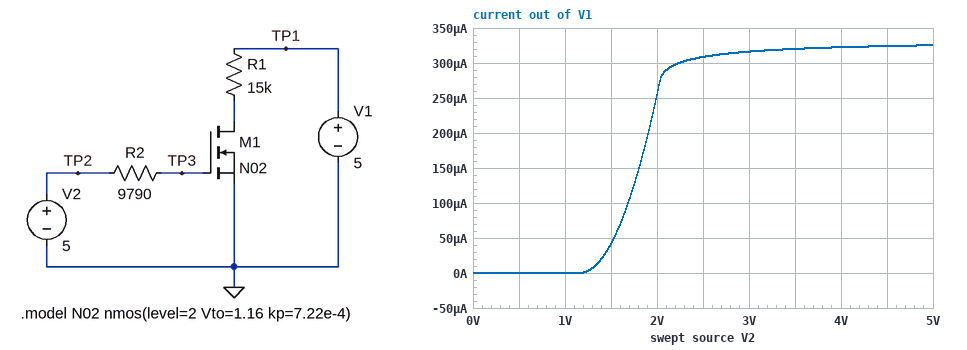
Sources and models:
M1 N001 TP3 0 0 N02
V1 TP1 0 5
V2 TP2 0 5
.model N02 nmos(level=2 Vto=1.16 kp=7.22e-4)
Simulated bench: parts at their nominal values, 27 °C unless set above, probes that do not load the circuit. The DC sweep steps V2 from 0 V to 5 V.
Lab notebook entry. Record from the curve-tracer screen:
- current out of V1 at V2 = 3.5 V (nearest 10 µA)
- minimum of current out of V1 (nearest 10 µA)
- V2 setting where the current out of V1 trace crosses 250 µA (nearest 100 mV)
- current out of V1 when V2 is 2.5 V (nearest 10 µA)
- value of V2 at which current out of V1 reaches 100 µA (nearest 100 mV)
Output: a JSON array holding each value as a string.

["320 µA", "0 A", "2.0 V", "310 µA", "1.7 V"]
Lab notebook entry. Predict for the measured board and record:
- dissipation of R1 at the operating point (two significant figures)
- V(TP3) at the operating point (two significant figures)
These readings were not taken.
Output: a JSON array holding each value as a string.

["1.6 mW", "5.0 V"]
